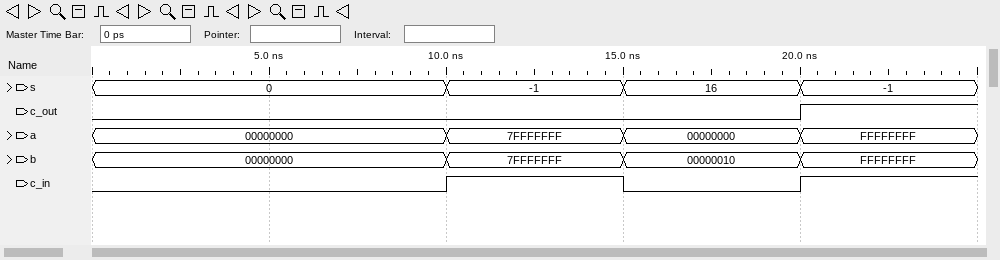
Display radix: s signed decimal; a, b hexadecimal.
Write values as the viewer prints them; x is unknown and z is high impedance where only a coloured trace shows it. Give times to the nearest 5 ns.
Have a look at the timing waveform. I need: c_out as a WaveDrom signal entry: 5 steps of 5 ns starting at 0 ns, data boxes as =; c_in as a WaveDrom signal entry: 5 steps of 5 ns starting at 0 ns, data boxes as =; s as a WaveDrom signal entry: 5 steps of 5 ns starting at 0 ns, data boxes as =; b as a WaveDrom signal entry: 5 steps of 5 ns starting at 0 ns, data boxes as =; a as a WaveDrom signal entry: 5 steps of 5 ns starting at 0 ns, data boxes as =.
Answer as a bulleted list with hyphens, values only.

- {name: 'c_out', wave: '0...1'}
- {name: 'c_in', wave: '0.101'}
- {name: 's', wave: '=.===', data: '0 -1 16 -1'}
- {name: 'b', wave: '=.===', data: '00000000 7FFFFFFF 00000010 FFFFFFFF'}
- {name: 'a', wave: '=.===', data: '00000000 7FFFFFFF 00000000 FFFFFFFF'}
